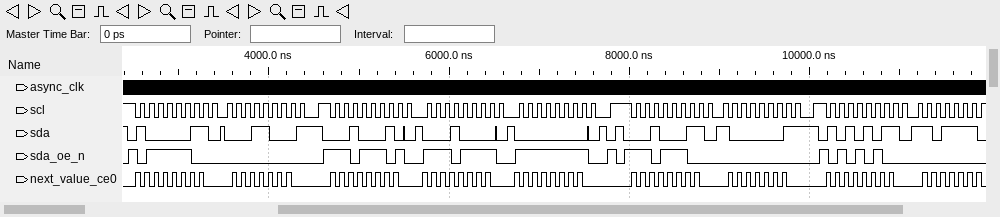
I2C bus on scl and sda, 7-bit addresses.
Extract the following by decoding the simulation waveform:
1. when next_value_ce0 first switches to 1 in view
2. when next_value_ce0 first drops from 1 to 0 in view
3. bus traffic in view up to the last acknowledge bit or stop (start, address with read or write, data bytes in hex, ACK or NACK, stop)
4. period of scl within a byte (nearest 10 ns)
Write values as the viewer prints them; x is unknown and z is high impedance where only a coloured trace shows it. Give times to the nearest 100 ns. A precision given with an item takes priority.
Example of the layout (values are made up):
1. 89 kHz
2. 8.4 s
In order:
1. 2500 ns
2. 2600 ns
3. start, address 41 read ACK, 18 NACK, repeated start, address 11 write ACK, 10 ACK, 00 ACK, stop, start, address 11 read ACK, 81 NACK, repeated start, address 55 read ACK
4. 100 ns
